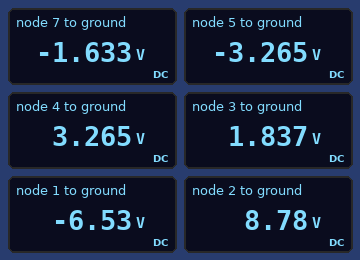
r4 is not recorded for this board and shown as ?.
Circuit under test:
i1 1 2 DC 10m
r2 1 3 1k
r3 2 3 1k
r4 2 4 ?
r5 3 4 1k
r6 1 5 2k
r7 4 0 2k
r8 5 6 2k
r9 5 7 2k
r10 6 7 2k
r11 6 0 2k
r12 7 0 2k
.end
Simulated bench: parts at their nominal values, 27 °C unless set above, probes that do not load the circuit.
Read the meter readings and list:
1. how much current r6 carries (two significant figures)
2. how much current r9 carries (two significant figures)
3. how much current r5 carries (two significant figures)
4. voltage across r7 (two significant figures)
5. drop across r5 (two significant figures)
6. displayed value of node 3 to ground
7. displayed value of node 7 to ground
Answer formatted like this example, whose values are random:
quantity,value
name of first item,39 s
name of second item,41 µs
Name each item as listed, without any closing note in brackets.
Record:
quantity,value
how much current r6 carries,1.6 mA
how much current r9 carries,820 µA
how much current r5 carries,1.4 mA
voltage across r7,3.3 V
drop across r5,1.4 V
displayed value of node 3 to ground,1.837 V
displayed value of node 7 to ground,-1.633 V
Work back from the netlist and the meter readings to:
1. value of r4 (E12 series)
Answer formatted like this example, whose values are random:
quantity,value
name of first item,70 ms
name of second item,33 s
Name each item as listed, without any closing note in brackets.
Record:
quantity,value
value of r4,1.8 kΩ
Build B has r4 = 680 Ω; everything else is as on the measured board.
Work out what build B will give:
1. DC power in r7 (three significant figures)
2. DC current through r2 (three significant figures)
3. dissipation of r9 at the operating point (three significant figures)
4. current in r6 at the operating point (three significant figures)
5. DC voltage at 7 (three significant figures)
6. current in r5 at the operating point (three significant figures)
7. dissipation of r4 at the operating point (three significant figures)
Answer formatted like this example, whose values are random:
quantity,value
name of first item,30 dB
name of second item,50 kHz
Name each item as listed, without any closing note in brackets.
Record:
quantity,value
DC power in r7,6.48 mW
DC current through r2,8.20 mA
dissipation of r9 at the operating point,1.62 mW
current in r6 at the operating point,1.80 mA
DC voltage at 7,-1.80 V
current in r5 at the operating point,2.60 mA
dissipation of r4 at the operating point,13.2 mW
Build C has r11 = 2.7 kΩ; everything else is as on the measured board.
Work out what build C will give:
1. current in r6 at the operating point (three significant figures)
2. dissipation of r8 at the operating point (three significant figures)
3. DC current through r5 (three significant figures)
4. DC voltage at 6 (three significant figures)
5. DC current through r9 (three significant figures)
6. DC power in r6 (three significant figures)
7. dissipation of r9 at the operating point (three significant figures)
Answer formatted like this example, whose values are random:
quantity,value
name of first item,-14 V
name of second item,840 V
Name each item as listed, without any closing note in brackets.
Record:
quantity,value
current in r6 at the operating point,1.60 mA
dissipation of r8 at the operating point,1.18 mW
DC current through r5,1.45 mA
DC voltage at 6,-1.91 V
DC current through r9,831 µA
DC power in r6,5.12 mW
dissipation of r9 at the operating point,1.38 mW
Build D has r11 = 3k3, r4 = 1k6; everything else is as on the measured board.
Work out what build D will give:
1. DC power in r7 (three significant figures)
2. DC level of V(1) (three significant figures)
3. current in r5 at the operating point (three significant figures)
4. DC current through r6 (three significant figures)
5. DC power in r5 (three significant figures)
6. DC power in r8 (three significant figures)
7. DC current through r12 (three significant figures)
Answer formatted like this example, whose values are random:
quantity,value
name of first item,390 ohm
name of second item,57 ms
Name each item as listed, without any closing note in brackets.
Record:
quantity,value
DC power in r7,5.12 mW
DC level of V(1),-6.82 V
current in r5 at the operating point,1.62 mA
DC current through r6,1.60 mA
DC power in r5,2.63 mW
DC power in r8,1.12 mW
DC current through r12,957 µA
